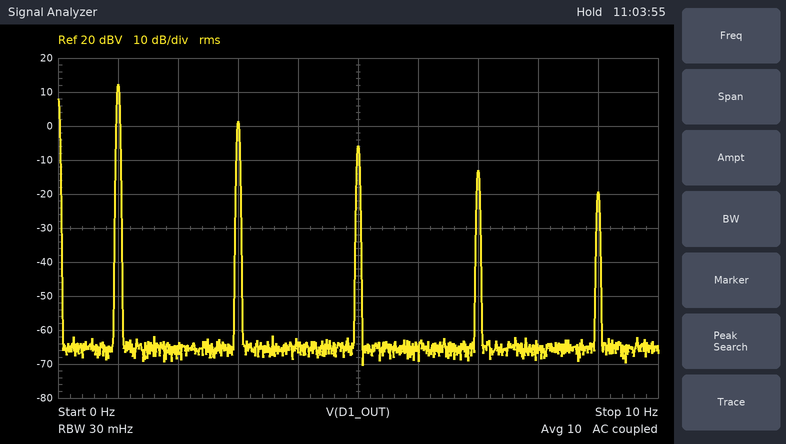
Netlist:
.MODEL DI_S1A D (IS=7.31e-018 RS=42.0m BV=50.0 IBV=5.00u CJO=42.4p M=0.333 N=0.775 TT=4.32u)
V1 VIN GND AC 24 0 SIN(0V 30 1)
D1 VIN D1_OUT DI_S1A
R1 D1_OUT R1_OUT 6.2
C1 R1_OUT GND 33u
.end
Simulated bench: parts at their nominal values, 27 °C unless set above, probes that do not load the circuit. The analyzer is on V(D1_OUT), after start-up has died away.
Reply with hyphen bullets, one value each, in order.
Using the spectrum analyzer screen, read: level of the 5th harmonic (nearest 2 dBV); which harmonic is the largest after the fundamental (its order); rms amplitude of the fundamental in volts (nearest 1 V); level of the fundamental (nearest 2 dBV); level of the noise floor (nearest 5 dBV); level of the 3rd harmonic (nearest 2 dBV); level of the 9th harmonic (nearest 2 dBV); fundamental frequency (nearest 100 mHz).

- -6 dBV
- 3
- 4 V
- 12 dBV
- -65 dBV
- 2 dBV
- -20 dBV
- 1.0 Hz
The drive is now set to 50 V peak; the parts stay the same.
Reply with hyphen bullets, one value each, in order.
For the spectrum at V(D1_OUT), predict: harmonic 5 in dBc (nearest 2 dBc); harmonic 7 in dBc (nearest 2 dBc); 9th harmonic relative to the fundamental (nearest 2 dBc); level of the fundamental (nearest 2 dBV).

- -28 dBc
- -32 dBc
- -38 dBc
- 26 dBV
